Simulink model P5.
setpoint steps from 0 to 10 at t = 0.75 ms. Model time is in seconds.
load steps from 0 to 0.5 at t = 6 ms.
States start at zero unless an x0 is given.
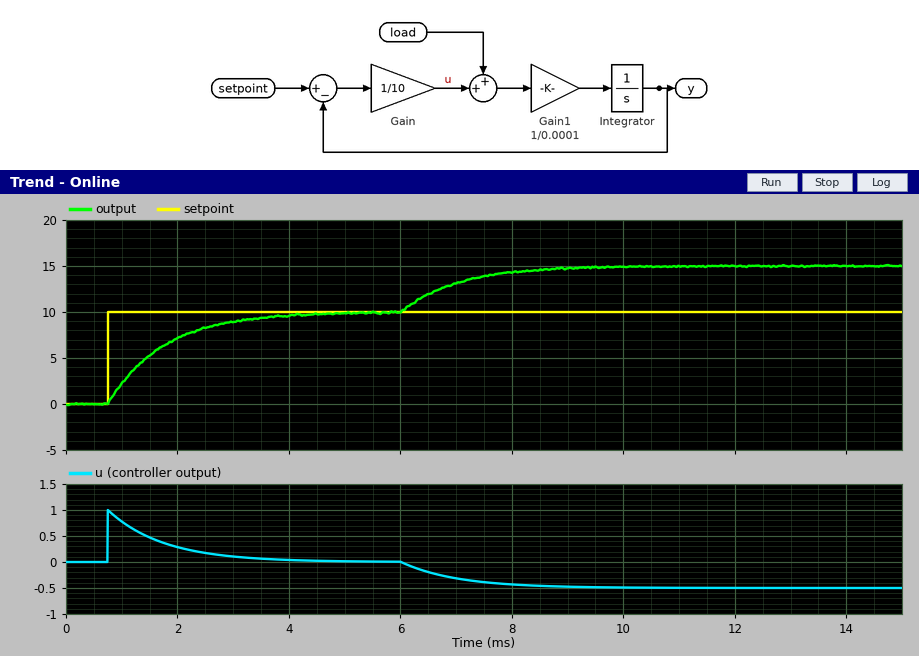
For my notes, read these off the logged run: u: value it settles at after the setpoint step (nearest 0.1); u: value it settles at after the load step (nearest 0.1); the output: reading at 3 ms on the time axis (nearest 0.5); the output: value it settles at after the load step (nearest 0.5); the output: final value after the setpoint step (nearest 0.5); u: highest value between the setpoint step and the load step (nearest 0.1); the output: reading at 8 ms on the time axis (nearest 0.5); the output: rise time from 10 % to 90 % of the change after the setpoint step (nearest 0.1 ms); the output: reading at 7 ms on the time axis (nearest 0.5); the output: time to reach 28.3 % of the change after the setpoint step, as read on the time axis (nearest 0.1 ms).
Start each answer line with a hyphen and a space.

- 0.0
- -0.5
- 9.0
- 15.0
- 10.0
- 1.0
- 14.5
- 2.2 ms
- 13.0
- 1.1 ms
